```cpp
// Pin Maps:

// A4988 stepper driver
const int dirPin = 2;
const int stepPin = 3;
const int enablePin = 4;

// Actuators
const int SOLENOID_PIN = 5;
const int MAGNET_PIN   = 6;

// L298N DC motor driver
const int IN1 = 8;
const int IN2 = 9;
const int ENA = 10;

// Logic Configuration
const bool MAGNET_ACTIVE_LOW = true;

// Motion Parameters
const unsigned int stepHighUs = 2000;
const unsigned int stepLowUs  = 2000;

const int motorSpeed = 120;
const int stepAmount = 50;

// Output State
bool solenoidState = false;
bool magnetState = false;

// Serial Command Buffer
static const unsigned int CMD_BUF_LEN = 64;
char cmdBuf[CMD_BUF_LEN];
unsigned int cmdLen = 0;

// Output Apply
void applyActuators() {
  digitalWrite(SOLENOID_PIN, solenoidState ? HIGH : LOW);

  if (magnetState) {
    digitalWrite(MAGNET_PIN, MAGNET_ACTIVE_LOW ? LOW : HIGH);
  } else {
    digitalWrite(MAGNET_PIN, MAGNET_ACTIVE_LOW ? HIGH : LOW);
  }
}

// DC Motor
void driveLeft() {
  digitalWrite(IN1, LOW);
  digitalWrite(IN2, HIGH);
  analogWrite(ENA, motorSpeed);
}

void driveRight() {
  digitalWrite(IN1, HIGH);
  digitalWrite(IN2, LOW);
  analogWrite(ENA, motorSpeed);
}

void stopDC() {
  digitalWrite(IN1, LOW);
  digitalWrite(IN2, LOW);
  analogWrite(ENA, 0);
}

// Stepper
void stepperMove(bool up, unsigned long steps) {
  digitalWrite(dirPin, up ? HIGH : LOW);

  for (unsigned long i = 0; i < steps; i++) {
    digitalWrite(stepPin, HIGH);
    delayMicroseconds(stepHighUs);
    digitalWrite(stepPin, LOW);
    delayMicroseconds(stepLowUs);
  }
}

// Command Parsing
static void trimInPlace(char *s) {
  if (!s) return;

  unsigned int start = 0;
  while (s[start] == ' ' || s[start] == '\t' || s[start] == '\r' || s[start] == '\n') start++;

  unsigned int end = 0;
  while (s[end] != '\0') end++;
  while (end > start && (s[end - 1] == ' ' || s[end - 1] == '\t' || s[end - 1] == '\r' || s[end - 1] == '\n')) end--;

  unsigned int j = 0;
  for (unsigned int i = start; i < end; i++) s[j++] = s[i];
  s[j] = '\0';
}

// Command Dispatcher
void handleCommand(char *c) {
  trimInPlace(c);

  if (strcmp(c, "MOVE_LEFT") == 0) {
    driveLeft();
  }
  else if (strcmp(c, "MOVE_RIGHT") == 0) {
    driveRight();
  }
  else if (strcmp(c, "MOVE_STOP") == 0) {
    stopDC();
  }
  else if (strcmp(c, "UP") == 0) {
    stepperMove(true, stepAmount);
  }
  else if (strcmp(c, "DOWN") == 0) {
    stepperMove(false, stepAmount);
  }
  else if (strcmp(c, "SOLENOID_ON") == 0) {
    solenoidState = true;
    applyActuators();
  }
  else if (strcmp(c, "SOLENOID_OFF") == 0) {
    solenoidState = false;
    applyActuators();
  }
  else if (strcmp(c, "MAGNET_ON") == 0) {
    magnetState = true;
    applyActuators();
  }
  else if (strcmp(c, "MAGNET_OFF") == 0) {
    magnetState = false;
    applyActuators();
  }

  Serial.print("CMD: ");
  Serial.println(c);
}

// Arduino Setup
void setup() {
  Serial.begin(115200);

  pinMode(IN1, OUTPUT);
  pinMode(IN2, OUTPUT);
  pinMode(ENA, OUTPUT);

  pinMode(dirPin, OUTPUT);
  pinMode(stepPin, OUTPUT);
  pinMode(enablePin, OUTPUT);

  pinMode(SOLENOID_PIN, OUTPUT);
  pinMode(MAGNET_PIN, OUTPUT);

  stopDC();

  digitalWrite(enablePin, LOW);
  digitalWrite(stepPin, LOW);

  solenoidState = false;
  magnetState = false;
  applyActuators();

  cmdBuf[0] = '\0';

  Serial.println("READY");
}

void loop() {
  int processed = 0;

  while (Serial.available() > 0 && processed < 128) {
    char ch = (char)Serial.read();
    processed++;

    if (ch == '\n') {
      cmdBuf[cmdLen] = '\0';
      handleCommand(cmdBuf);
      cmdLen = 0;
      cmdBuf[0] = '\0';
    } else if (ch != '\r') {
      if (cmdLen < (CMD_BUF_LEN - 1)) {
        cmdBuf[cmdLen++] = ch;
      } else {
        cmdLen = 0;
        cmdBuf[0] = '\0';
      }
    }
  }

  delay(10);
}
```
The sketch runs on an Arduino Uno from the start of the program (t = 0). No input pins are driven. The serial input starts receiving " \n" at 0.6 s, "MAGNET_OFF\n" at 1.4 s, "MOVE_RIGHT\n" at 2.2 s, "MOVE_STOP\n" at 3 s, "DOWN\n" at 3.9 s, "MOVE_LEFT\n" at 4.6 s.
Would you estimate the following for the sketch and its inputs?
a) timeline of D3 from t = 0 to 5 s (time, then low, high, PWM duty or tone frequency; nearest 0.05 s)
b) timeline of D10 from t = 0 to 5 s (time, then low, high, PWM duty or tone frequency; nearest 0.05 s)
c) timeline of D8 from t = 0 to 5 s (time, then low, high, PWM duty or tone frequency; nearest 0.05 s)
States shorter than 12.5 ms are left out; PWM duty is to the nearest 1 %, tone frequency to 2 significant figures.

0 s low; 3.9 s tone 250 Hz; 4.1 s low
0 s low; 2.2 s PWM 47 %; 3 s low; 4.6 s PWM 47 %
0 s low; 2.2 s high; 3 s low
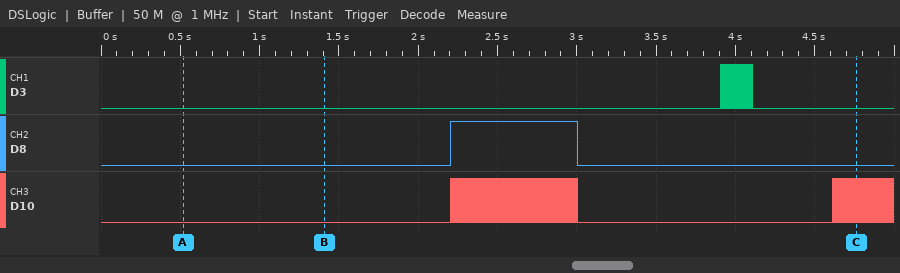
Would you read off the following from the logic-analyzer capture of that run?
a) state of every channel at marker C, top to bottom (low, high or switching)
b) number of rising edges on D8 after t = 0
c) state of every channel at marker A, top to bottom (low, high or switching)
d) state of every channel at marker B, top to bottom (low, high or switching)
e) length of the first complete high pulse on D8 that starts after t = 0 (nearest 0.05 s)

D3 low, D8 low, D10 switching
1
D3 low, D8 low, D10 low
D3 low, D8 low, D10 low
0.80 s
